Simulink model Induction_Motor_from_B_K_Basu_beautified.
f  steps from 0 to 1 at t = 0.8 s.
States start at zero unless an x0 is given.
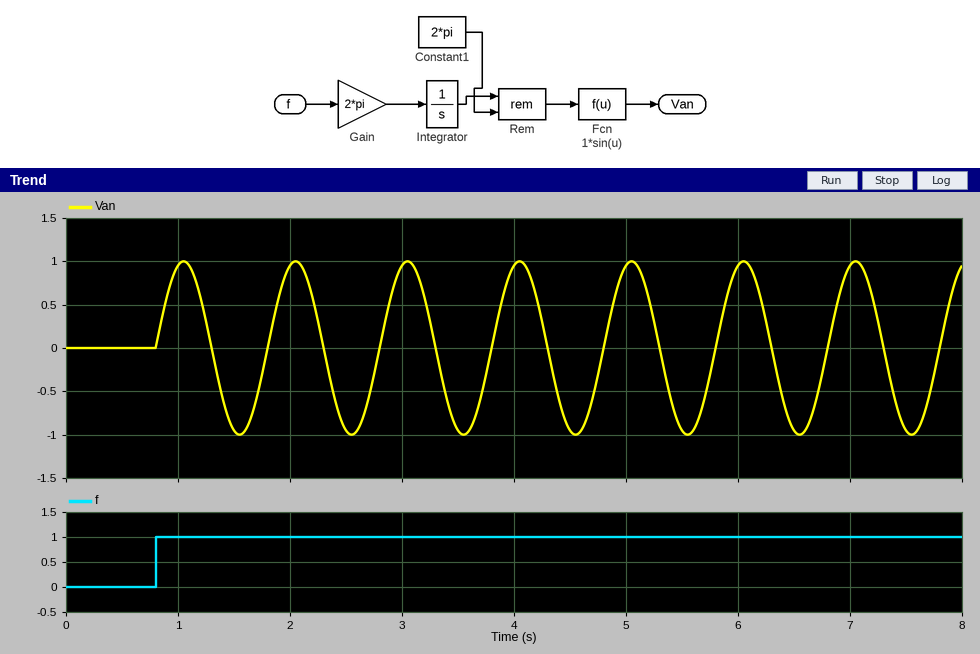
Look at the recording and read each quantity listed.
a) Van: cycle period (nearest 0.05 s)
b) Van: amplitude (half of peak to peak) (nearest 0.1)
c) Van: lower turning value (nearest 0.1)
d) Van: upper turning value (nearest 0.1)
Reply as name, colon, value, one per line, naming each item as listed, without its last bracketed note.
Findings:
Van: cycle period: 1.00 s
Van: amplitude (half of peak to peak): 1.0
Van: lower turning value: -1.0
Van: upper turning value: 1.0
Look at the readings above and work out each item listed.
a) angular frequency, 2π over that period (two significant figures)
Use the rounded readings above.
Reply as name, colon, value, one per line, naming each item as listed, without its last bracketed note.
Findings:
angular frequency, 2π over that period: 6.3 rad/s
